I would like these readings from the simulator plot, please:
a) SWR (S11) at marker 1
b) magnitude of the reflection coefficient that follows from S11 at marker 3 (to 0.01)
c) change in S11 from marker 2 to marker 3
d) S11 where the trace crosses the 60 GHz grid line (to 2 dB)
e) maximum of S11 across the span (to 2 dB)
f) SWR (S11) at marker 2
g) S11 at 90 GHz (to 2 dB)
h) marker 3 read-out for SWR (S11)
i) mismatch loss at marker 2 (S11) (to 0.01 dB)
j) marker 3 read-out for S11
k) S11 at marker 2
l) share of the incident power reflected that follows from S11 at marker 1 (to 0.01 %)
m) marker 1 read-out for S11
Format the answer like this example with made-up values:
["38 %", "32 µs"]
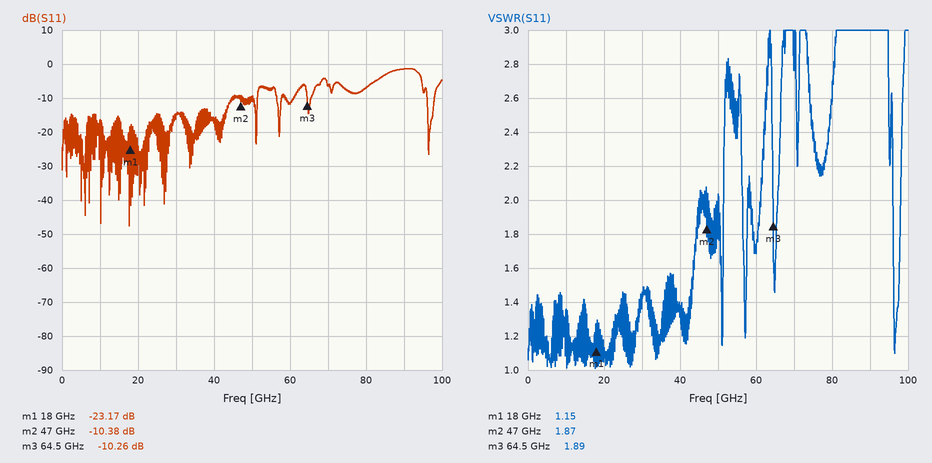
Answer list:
["1.15", "0.31", "0.12 dB", "-12 dB", "-2 dB", "1.87", "-2 dB", "1.89", "0.42 dB", "-10.26 dB", "-10.38 dB", "0.48 %", "-23.17 dB"]
